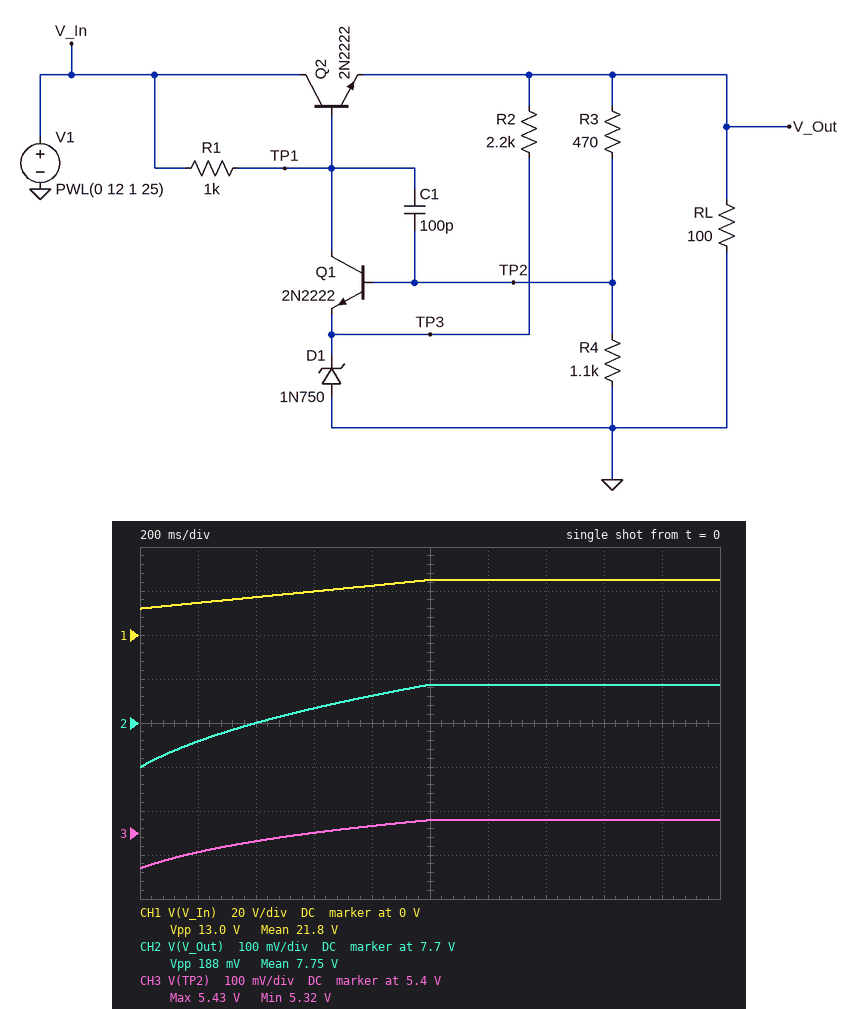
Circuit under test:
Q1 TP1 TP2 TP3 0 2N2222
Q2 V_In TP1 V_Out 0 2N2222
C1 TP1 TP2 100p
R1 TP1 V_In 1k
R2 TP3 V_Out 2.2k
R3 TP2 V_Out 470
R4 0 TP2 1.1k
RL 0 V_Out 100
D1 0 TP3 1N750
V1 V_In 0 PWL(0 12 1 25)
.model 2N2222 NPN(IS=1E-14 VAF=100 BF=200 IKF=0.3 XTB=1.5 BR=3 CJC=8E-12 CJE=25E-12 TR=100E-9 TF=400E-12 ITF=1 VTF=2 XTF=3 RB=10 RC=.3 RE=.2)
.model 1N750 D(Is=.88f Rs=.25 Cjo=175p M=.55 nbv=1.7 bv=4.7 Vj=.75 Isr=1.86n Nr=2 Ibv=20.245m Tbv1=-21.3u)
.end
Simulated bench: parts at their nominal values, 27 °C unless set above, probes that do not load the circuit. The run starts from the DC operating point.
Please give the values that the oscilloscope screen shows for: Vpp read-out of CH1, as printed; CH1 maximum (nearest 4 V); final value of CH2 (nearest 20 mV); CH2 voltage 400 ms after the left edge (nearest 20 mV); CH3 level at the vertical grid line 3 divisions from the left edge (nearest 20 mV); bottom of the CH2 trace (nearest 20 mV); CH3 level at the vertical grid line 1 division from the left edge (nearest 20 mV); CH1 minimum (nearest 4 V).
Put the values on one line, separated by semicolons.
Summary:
13.0 V; 24 V; 7.78 V; 7.70 V; 5.40 V; 7.60 V; 5.36 V; 12 V
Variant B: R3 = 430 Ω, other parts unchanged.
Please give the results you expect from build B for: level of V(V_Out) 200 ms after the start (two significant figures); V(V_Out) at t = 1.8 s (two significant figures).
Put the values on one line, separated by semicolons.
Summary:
7.5 V; 7.6 V
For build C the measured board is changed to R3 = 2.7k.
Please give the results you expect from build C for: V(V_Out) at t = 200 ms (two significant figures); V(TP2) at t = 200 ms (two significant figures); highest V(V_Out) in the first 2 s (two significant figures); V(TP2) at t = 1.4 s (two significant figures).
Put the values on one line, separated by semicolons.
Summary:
13 V; 3.7 V; 19 V; 5.4 V
